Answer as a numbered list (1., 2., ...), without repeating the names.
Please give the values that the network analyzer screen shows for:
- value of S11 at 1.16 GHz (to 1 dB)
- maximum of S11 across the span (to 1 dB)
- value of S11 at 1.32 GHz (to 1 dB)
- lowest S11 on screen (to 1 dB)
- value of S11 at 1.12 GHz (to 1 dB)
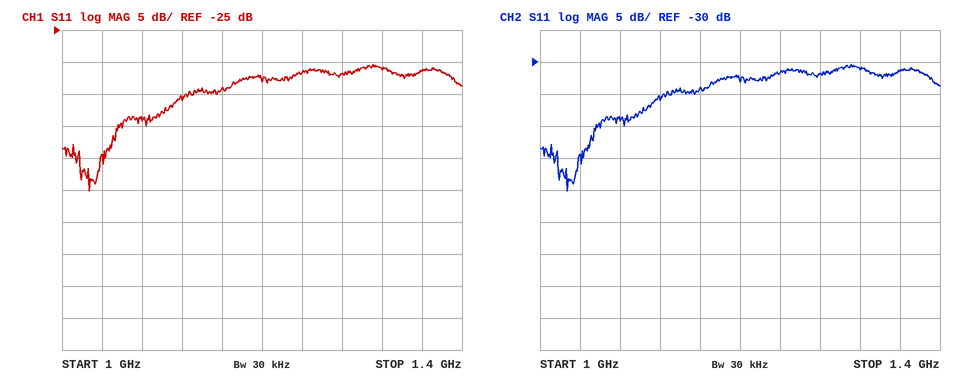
1. -34 dB
2. -30 dB
3. -31 dB
4. -50 dB
5. -36 dB
